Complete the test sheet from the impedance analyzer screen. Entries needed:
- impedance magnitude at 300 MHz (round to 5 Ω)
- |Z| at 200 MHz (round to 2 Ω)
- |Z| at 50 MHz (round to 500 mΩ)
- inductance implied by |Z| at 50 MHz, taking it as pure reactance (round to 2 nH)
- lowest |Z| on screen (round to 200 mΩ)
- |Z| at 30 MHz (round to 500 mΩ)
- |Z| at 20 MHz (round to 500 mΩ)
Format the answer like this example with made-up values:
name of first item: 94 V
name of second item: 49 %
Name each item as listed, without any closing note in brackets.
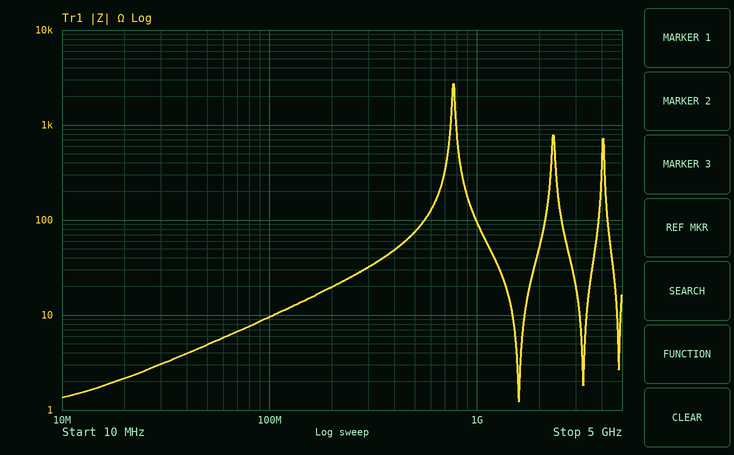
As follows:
impedance magnitude at 300 MHz: 30 Ω
|Z| at 200 MHz: 20 Ω
|Z| at 50 MHz: 5.0 Ω
inductance implied by |Z| at 50 MHz, taking it as pure reactance: 16 nH
lowest |Z| on screen: 1.2 Ω
|Z| at 30 MHz: 3.0 Ω
|Z| at 20 MHz: 2.0 Ω
